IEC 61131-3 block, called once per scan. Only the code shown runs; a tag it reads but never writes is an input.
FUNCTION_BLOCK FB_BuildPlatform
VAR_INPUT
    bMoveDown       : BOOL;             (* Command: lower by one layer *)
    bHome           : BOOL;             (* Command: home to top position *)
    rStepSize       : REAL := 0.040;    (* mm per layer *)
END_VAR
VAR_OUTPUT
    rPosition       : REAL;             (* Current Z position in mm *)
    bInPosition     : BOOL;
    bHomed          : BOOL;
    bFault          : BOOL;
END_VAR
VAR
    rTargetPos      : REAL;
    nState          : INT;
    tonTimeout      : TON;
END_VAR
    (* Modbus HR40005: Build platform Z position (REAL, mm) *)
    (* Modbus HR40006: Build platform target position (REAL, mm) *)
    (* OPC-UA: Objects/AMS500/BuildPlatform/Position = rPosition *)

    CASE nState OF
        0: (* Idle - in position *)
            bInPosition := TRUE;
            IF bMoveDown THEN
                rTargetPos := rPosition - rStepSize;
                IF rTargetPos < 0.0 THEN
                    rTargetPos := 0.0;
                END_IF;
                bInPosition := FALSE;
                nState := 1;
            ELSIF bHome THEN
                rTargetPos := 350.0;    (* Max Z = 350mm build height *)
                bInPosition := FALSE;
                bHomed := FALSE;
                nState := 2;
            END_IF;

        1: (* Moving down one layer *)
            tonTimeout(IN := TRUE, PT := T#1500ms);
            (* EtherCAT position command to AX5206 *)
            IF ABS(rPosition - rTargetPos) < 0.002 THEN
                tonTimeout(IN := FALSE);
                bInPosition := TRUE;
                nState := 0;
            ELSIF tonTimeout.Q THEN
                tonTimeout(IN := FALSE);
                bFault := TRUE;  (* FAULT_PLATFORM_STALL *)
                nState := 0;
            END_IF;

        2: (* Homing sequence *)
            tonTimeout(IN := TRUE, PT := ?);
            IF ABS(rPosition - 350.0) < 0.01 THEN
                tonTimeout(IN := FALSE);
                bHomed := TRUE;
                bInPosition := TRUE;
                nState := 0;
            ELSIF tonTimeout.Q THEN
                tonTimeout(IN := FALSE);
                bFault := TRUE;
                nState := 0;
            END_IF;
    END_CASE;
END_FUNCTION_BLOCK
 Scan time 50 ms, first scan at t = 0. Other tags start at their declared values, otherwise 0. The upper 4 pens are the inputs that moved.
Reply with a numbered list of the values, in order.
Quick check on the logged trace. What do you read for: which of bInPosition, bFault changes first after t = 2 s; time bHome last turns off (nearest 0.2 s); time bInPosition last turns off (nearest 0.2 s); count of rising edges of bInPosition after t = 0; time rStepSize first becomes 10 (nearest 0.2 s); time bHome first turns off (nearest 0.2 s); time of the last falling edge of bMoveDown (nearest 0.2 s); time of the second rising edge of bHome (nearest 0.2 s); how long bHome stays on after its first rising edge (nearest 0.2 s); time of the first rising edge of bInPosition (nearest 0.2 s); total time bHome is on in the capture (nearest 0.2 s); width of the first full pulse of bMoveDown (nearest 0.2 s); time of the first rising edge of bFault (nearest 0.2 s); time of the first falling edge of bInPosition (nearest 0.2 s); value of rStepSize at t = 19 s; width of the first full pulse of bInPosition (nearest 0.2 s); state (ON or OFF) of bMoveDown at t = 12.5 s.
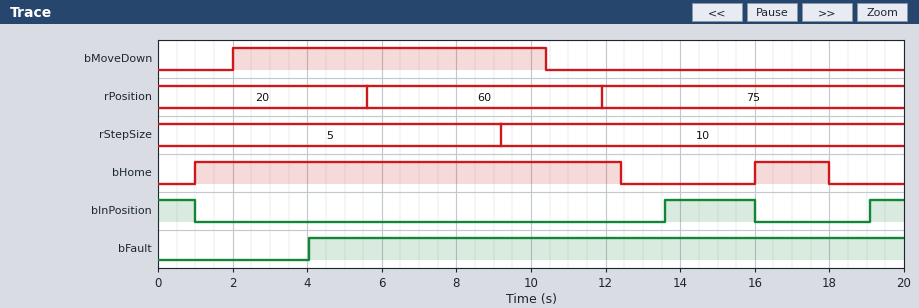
1. bFault
2. 18.0 s
3. 16.0 s
4. 2
5. 9.2 s
6. 12.4 s
7. 10.4 s
8. 16.0 s
9. 11.4 s
10. 13.6 s
11. 13.4 s
12. 8.4 s
13. 4.0 s
14. 1.0 s
15. 10
16. 2.4 s
17. OFF
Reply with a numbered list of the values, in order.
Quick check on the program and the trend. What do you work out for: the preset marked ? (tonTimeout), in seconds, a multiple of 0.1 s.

1. 3.0 s
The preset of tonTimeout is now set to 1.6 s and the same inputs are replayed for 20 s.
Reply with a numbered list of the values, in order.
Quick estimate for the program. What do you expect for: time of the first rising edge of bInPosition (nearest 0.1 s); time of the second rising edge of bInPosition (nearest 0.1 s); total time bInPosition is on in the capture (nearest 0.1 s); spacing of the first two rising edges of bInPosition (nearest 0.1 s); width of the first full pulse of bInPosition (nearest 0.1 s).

1. 12.4 s
2. 19.4 s
3. 5.2 s
4. 7.0 s
5. 3.6 s
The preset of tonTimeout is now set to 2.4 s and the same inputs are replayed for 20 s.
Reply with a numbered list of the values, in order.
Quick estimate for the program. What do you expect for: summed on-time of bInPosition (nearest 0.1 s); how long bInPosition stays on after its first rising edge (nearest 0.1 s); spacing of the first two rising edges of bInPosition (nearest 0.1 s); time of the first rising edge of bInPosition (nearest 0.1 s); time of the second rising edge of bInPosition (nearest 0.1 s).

1. 4.5 s
2. 2.0 s
3. 4.5 s
4. 14.0 s
5. 18.5 s
